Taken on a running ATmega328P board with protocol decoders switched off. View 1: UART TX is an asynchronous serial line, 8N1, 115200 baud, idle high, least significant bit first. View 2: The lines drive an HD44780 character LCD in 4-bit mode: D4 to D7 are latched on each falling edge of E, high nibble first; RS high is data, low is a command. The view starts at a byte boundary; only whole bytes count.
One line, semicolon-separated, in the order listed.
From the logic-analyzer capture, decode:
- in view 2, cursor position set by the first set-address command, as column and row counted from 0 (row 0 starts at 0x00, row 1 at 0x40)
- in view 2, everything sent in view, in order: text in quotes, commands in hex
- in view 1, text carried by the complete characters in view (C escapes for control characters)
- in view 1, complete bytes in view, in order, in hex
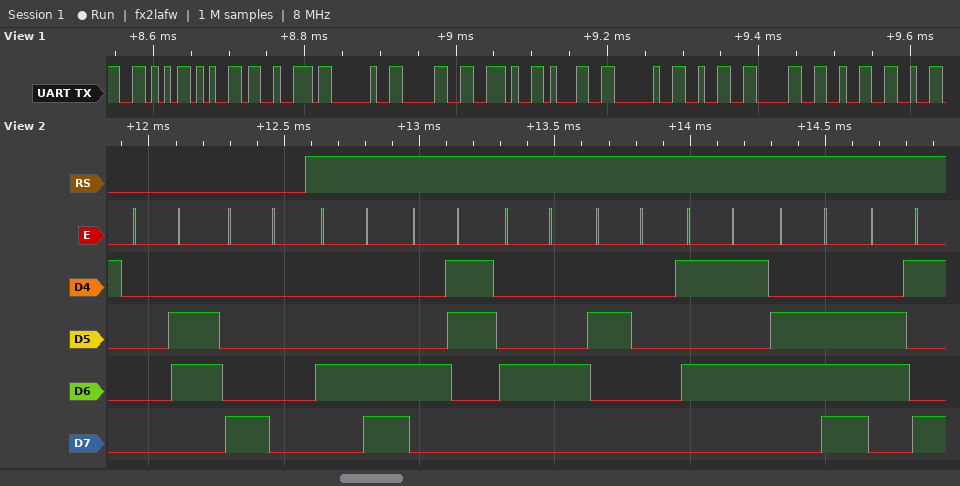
column 0, row 0; 0x06 0x80 "LCD Uni"; "Ver 0.1 202"; 56 65 72 20 30 2E 31 20 32 30 32
